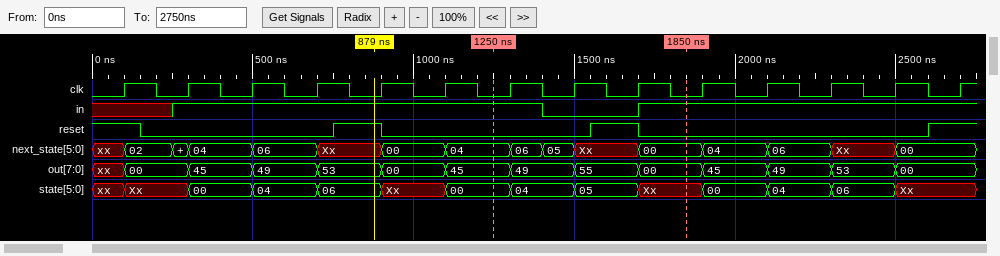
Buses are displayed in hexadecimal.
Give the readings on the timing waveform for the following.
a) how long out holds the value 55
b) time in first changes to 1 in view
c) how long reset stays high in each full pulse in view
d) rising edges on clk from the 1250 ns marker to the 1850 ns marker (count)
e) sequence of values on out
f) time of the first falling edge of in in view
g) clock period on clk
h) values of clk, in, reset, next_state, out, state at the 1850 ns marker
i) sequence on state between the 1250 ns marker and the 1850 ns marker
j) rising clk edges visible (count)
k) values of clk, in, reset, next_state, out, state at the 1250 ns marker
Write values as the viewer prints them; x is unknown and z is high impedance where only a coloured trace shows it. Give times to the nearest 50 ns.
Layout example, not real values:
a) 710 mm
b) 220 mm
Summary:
a) 200 ns
b) 250 ns
c) 150 ns, 150 ns
d) 3
e) xx, 00, 45, 49, 53, 00, 45, 49, 55, 00, 45, 49, 53, 00
f) 1400 ns
g) 200 ns
h) clk=0, in=1, reset=0, next_state=00, out=00, state=Xx
i) 00, 04, 05, Xx
j) 14
k) clk=0, in=1, reset=0, next_state=04, out=45, state=00
